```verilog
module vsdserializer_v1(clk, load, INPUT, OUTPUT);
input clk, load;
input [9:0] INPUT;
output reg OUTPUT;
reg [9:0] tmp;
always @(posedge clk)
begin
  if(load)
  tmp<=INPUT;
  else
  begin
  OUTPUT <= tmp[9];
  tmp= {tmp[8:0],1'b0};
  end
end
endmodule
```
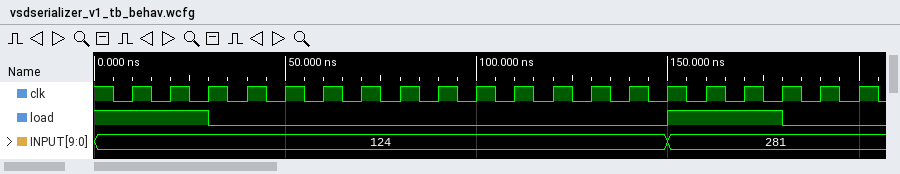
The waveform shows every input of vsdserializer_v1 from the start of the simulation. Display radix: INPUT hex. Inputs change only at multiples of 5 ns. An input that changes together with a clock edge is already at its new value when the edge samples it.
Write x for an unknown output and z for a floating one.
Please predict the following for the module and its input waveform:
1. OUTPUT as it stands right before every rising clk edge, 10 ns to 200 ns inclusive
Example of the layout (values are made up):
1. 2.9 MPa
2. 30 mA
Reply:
1. x x x 0 1 0 0 1 0 0 1 0 0 0 0 0 0 0 1 0
